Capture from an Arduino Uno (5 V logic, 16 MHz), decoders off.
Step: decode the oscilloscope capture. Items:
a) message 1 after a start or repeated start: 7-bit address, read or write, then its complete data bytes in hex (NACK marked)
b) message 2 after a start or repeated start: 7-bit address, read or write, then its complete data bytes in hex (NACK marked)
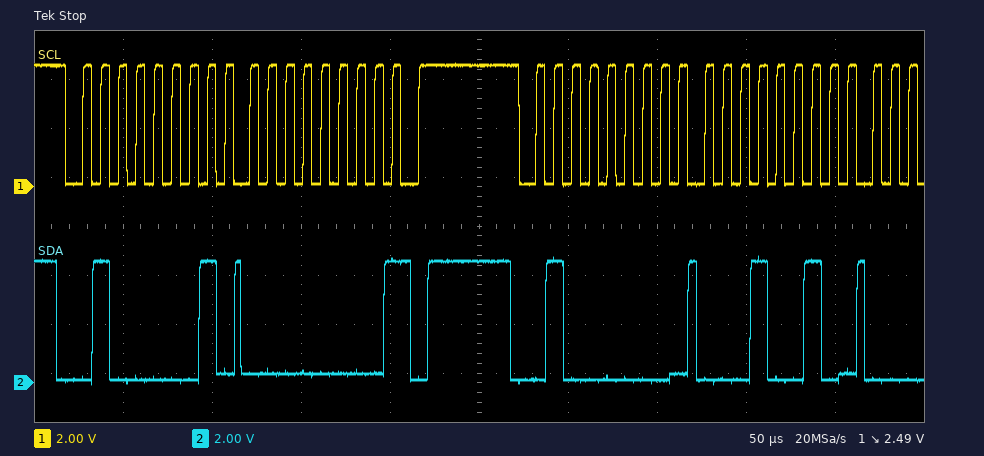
0x20 read: 00 NACK
0x20 write: 12
